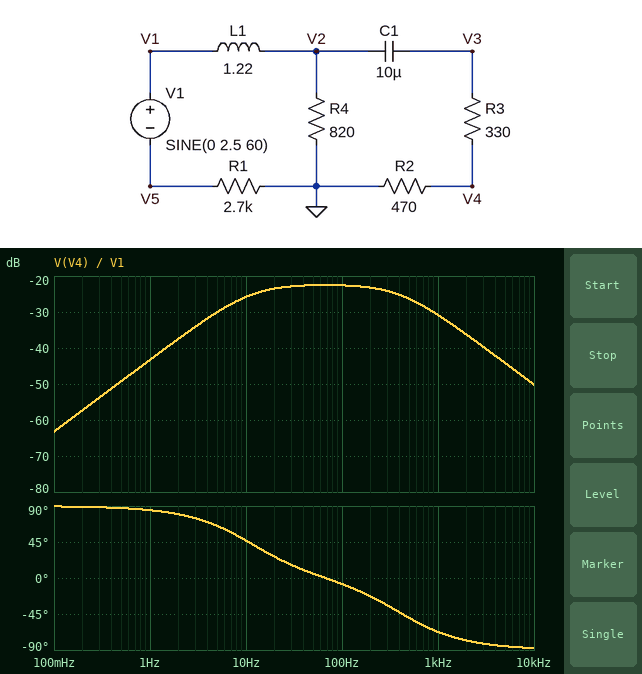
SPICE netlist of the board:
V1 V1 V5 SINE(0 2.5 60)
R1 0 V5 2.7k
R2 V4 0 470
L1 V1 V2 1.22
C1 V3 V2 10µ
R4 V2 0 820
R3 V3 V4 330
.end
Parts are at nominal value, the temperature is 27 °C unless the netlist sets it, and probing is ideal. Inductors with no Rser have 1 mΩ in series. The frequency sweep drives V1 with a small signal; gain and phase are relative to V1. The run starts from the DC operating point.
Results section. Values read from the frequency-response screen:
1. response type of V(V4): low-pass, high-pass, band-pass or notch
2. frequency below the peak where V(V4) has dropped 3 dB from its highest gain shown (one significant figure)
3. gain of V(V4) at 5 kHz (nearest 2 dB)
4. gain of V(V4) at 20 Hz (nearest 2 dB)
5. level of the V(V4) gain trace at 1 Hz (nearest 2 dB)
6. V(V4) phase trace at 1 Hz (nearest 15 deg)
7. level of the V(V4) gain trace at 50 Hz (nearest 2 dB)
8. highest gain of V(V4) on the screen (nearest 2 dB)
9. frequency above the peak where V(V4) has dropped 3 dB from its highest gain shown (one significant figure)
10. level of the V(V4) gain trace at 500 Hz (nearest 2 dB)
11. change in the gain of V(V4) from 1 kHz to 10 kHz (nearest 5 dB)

band-pass
10 Hz
-44 dB
-24 dB
-44 dB
90 deg
-22 dB
-22 dB
400 Hz
-26 dB
-20 dB
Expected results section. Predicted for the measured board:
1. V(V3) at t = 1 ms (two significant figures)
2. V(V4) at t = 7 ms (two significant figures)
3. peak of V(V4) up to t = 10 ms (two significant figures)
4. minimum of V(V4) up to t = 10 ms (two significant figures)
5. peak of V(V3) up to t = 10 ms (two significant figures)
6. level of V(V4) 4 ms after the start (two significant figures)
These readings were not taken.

75 mV
62 mV
160 mV
-130 mV
270 mV
160 mV
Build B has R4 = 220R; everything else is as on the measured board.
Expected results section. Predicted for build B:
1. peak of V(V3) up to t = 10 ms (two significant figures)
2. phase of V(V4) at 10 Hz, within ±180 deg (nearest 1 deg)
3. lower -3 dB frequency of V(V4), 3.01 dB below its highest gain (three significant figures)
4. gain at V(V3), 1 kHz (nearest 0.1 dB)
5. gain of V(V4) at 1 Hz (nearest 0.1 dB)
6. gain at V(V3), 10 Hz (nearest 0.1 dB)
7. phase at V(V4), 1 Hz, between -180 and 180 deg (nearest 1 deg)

120 mV
56 deg
14.7 Hz
-33.5 dB
-53.1 dB
-29.9 dB
86 deg
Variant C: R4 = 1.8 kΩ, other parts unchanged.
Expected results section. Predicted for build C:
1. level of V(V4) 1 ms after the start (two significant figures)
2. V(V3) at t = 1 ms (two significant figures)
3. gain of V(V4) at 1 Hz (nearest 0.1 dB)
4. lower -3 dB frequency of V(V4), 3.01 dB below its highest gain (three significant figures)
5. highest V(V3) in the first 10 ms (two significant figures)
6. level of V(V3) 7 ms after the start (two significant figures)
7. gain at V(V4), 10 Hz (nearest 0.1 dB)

59 mV
100 mV
-38.6 dB
8.19 Hz
370 mV
160 mV
-22.3 dB
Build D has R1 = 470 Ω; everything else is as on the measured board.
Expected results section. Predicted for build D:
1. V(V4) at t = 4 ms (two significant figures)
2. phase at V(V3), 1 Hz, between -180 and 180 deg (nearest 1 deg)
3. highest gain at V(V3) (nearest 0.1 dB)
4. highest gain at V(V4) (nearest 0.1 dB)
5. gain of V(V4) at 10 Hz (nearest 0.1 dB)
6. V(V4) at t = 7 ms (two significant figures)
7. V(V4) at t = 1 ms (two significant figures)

460 mV
86 deg
-7.4 dB
-12.0 dB
-16.1 dB
320 mV
71 mV
